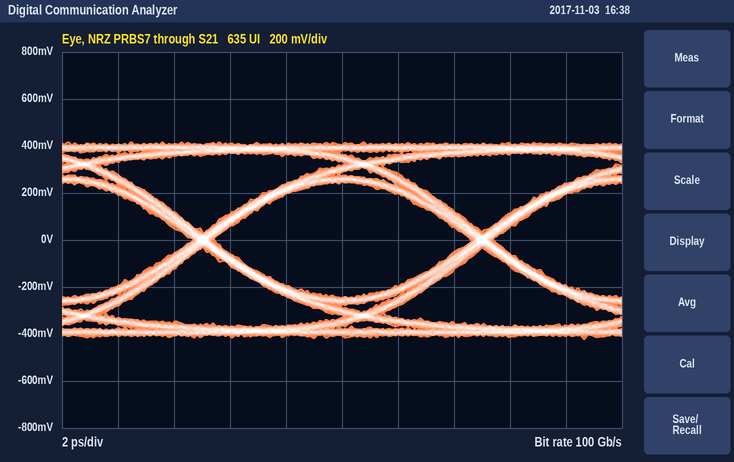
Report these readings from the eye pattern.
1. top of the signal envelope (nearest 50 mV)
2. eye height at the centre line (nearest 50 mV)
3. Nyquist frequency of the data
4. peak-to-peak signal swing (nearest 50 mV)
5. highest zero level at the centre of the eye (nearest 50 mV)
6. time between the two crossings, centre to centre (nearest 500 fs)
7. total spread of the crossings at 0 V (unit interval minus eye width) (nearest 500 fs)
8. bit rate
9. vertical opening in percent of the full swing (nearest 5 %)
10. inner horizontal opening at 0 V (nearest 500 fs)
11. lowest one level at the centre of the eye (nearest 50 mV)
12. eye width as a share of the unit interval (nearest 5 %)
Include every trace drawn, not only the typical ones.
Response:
400 mV
500 mV
50 GHz
850 mV
-250 mV
10.0 ps
1.0 ps
100 Gb/s
60 %
9.0 ps
250 mV
90 %
